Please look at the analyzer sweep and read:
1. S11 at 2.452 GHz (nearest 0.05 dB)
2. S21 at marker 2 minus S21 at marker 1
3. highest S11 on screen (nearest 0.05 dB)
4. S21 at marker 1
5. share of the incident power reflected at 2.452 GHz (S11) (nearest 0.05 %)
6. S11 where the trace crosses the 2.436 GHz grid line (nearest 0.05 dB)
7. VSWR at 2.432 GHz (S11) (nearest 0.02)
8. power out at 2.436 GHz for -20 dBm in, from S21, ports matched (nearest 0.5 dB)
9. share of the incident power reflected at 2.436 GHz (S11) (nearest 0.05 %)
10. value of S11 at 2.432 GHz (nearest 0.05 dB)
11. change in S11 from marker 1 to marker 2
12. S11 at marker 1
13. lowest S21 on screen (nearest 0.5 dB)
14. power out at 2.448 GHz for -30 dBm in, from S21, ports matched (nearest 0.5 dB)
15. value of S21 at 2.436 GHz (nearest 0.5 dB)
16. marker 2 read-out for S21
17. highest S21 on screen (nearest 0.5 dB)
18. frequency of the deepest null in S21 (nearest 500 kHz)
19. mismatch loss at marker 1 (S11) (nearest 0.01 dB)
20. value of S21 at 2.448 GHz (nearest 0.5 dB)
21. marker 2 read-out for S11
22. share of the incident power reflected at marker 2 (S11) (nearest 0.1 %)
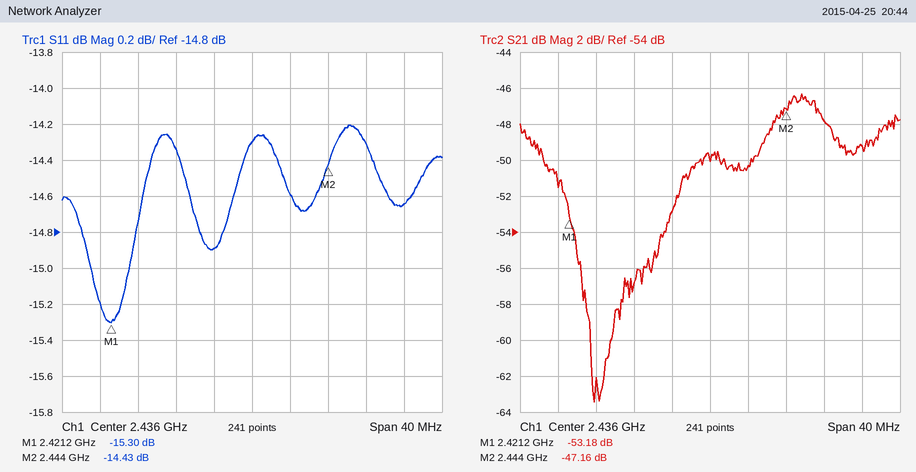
-14.65 dB
6.02 dB
-14.20 dB
-53.18 dB
3.45 %
-14.30 dB
1.44
-70.0 dBm
3.70 %
-14.90 dB
0.87 dB
-15.30 dB
-63.5 dB
-78.0 dBm
-50.0 dB
-47.16 dB
-46.5 dB
2.4240 GHz
0.13 dB
-48.0 dB
-14.43 dB
3.6 %
